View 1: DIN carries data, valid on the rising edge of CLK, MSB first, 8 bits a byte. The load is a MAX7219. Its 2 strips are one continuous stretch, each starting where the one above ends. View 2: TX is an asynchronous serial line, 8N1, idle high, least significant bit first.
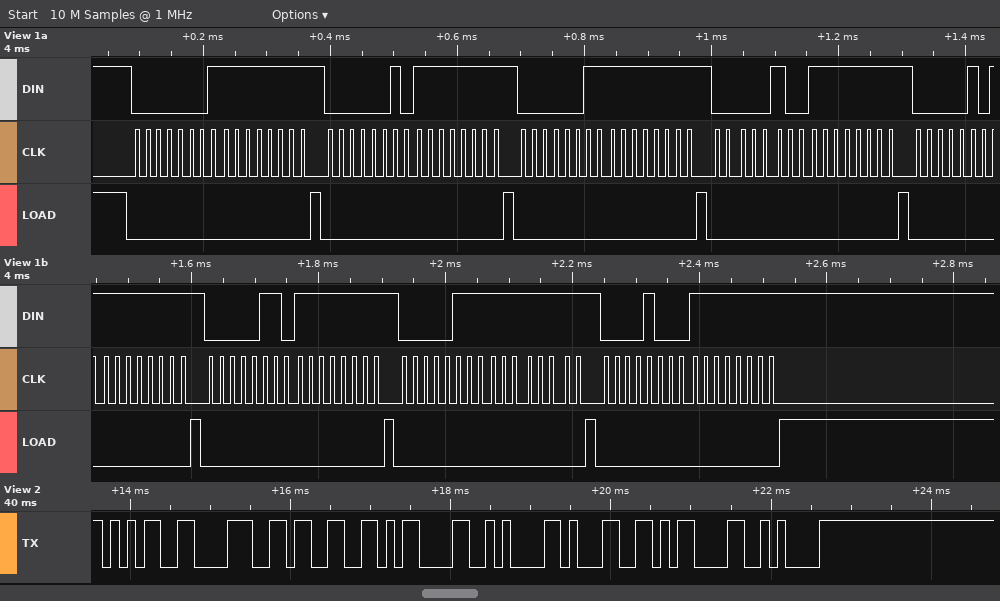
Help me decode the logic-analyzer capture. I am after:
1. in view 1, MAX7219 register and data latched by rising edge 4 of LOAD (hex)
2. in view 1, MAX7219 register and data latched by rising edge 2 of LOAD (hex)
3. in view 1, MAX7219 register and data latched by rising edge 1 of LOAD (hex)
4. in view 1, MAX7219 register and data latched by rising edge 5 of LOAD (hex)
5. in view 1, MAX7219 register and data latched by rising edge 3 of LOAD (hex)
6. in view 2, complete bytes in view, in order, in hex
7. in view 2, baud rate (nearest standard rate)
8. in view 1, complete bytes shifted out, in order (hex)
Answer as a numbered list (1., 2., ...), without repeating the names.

1. register 0x4, data 0xFF
2. register 0x2, data 0xFF
3. register 0x1, data 0xFF
4. register 0x5, data 0xFF
5. register 0x3, data 0xFF
6. 35 38 33 0D 0A 31 0D 0A
7. 9600 baud
8. 0x01 0xFF 0x02 0xFF 0x03 0xFF 0x04 0xFF 0x05 0xFF 0x06 0xFF 0x07 0xFF 0x08 0xFF
